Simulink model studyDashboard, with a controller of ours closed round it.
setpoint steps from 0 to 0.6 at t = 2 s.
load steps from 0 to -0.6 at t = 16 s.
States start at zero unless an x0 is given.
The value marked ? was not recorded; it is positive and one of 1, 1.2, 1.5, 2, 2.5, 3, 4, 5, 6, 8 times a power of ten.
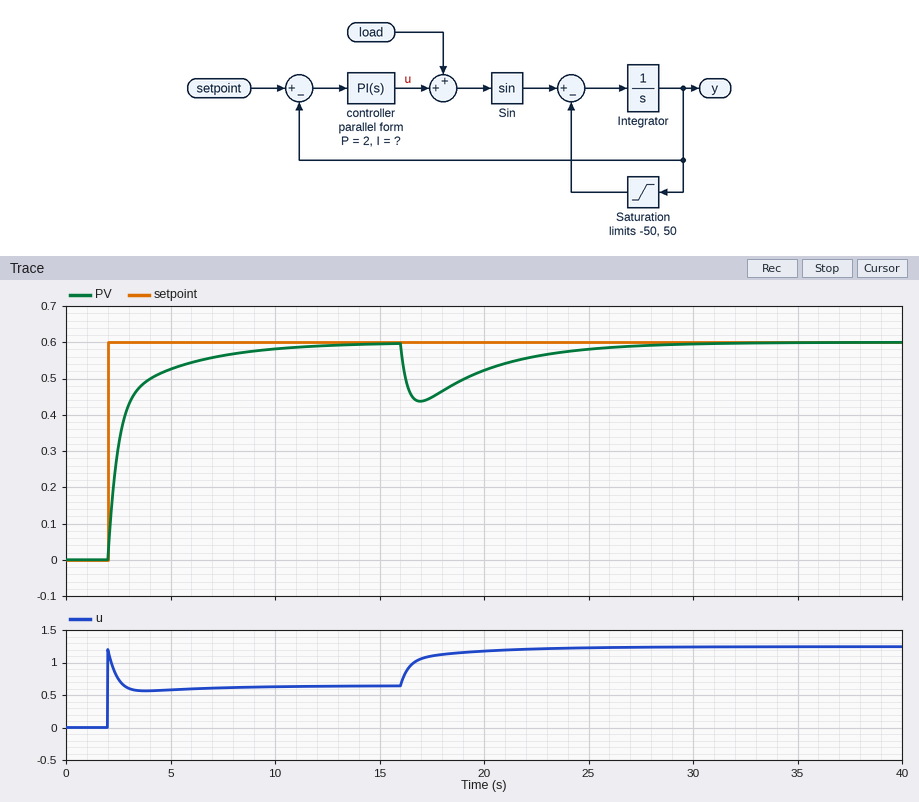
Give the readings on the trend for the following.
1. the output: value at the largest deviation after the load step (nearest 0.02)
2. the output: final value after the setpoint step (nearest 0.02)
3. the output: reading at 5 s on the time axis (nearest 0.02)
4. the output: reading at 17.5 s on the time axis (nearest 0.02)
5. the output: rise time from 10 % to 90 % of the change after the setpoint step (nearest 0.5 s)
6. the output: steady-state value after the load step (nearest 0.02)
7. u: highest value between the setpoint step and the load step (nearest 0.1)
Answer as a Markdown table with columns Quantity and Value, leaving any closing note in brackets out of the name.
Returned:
| Quantity | Value |
|---|---|
| the output: value at the largest deviation after the load step | 0.44 |
| the output: final value after the setpoint step | 0.60 |
| the output: reading at 5 s on the time axis | 0.52 |
| the output: reading at 17.5 s on the time axis | 0.44 |
| the output: rise time from 10 % to 90 % of the change after the setpoint step | 3.5 s |
| the output: steady-state value after the load step | 0.60 |
| u: highest value between the setpoint step and the load step | 1.2 |
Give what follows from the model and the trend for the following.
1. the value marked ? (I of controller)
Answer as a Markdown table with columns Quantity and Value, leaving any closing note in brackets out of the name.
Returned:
| Quantity | Value |
|---|---|
| the value marked ? | 0.8 |
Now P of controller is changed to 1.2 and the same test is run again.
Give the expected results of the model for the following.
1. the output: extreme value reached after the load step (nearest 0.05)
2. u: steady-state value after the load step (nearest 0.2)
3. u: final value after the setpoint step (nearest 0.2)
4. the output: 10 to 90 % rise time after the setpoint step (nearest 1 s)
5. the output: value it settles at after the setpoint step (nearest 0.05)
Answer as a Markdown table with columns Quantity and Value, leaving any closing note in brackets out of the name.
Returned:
| Quantity | Value |
|---|---|
| the output: extreme value reached after the load step | 0.40 |
| u: steady-state value after the load step | 1.2 |
| u: final value after the setpoint step | 0.6 |
| the output: 10 to 90 % rise time after the setpoint step | 3 s |
| the output: value it settles at after the setpoint step | 0.60 |
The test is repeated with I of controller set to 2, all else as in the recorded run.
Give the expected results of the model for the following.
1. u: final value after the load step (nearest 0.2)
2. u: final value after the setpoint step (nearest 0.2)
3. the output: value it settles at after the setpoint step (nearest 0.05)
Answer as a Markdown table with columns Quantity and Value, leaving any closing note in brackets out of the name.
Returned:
| Quantity | Value |
|---|---|
| u: final value after the load step | 1.2 |
| u: final value after the setpoint step | 0.6 |
| the output: value it settles at after the setpoint step | 0.60 |
